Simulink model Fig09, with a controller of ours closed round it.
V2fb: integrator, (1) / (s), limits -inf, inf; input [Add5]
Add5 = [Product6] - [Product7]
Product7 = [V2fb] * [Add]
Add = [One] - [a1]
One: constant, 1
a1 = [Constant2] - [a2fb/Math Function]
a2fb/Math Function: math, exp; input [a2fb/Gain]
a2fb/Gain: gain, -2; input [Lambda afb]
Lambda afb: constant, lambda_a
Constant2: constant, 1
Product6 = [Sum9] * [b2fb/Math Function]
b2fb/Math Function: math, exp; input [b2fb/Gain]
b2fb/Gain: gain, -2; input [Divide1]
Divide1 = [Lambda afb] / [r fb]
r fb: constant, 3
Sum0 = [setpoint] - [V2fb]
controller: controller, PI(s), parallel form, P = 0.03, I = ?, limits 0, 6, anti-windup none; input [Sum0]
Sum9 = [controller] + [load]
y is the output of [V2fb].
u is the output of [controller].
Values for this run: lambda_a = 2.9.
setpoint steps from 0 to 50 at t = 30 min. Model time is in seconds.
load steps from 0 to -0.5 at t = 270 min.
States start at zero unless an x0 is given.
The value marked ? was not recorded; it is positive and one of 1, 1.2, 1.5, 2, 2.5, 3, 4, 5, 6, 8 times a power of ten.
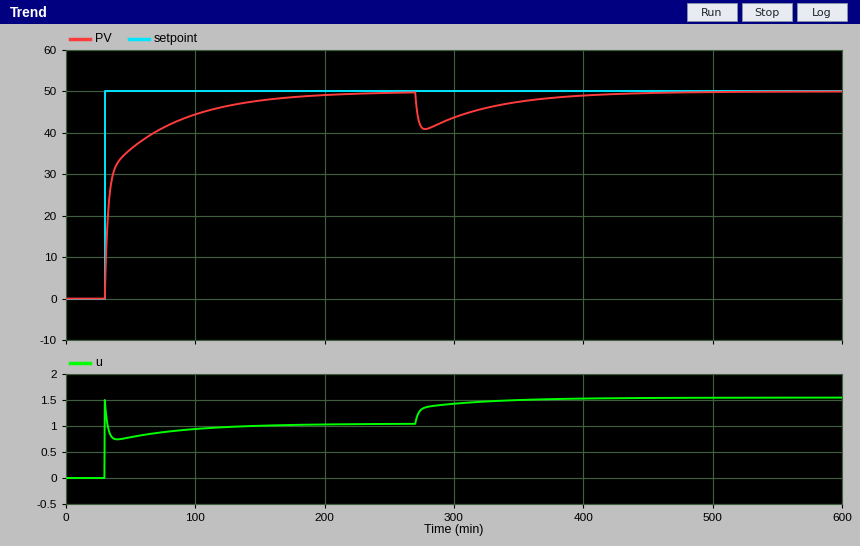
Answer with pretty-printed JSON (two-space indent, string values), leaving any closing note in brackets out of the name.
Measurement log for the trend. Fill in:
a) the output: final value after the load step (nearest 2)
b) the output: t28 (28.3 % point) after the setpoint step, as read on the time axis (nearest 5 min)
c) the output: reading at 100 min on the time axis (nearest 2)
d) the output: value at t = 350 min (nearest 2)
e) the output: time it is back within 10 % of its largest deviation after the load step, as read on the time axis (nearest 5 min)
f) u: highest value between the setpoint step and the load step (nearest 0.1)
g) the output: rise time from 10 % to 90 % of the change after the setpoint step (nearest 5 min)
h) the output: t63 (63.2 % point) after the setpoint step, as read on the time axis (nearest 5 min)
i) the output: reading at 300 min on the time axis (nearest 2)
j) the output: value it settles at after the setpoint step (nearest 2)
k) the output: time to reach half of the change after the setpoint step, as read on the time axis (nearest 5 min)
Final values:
{
  "the output: final value after the load step": "50",
  "the output: t28 (28.3 % point) after the setpoint step, as read on the time axis": "30 min",
  "the output: reading at 100 min on the time axis": "44",
  "the output: value at t = 350 min": "48",
  "the output: time it is back within 10 % of its largest deviation after the load step, as read on the time axis": "405 min",
  "u: highest value between the setpoint step and the load step": "1.5",
  "the output: rise time from 10 % to 90 % of the change after the setpoint step": "75 min",
  "the output: t63 (63.2 % point) after the setpoint step, as read on the time axis": "40 min",
  "the output: reading at 300 min on the time axis": "44",
  "the output: value it settles at after the setpoint step": "50",
  "the output: time to reach half of the change after the setpoint step, as read on the time axis": "35 min"
}
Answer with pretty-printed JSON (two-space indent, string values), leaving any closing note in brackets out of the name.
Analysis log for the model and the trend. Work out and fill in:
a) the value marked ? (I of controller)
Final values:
{
  "the value marked ?": "1.5e-05"
}
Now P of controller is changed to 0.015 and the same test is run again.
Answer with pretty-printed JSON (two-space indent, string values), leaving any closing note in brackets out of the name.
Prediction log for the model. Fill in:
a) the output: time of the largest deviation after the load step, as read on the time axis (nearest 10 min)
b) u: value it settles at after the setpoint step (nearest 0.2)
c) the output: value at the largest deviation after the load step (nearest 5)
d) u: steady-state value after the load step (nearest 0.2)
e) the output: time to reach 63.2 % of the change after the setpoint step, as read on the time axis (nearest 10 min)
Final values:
{
  "the output: time of the largest deviation after the load step, as read on the time axis": "280 min",
  "u: value it settles at after the setpoint step": "1.0",
  "the output: value at the largest deviation after the load step": "40",
  "u: steady-state value after the load step": "1.6",
  "the output: time to reach 63.2 % of the change after the setpoint step, as read on the time axis": "50 min"
}
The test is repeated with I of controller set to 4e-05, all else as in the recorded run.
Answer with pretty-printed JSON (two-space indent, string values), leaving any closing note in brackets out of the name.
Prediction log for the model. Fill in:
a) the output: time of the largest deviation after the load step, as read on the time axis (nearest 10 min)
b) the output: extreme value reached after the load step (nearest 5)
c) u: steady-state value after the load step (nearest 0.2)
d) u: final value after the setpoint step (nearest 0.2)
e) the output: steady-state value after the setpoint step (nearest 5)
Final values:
{
  "the output: time of the largest deviation after the load step, as read on the time axis": "280 min",
  "the output: extreme value reached after the load step": "40",
  "u: steady-state value after the load step": "1.6",
  "u: final value after the setpoint step": "1.0",
  "the output: steady-state value after the setpoint step": "50"
}
